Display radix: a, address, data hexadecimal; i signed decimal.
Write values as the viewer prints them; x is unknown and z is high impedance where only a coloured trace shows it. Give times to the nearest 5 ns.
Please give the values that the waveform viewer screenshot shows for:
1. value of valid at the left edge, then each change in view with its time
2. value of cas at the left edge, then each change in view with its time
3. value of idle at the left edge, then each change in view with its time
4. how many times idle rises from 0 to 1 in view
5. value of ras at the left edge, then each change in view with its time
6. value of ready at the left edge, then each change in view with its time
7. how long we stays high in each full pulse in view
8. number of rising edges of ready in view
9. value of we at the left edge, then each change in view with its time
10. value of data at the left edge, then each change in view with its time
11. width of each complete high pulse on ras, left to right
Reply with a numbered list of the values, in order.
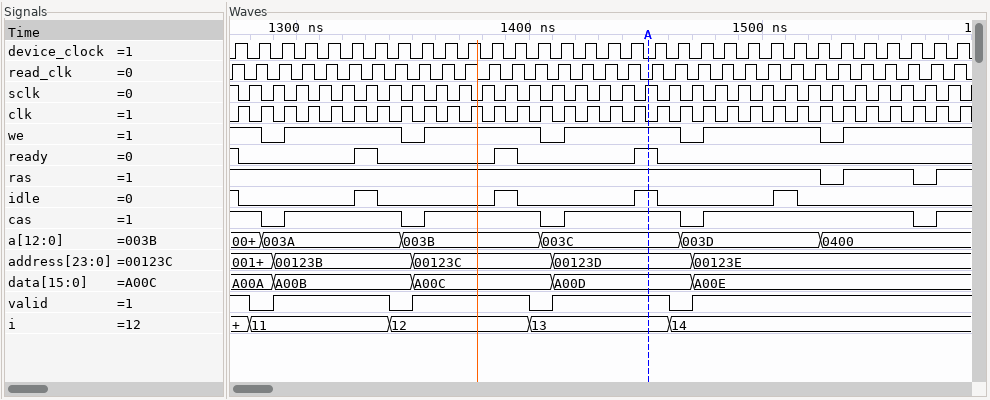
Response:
1. 1, 0 at 1280 ns, 1 at 1290 ns, 0 at 1340 ns, 1 at 1350 ns, 0 at 1400 ns, 1 at 1410 ns, 0 at 1460 ns, 1 at 1470 ns
2. 1, 0 at 1285 ns, 1 at 1295 ns, 0 at 1345 ns, 1 at 1355 ns, 0 at 1405 ns, 1 at 1415 ns, 0 at 1465 ns, 1 at 1475 ns, 0 at 1565 ns, 1 at 1575 ns
3. 1, 0 at 1275 ns, 1 at 1325 ns, 0 at 1335 ns, 1 at 1385 ns, 0 at 1395 ns, 1 at 1445 ns, 0 at 1455 ns, 1 at 1505 ns, 0 at 1515 ns
4. 4
5. 1, 0 at 1525 ns, 1 at 1535 ns, 0 at 1565 ns, 1 at 1575 ns
6. 1, 0 at 1275 ns, 1 at 1325 ns, 0 at 1335 ns, 1 at 1385 ns, 0 at 1395 ns, 1 at 1445 ns, 0 at 1455 ns
7. 50 ns, 50 ns, 50 ns, 50 ns
8. 3
9. 1, 0 at 1285 ns, 1 at 1295 ns, 0 at 1345 ns, 1 at 1355 ns, 0 at 1405 ns, 1 at 1415 ns, 0 at 1465 ns, 1 at 1475 ns, 0 at 1525 ns, 1 at 1535 ns
10. A00A, A00B at 1290 ns, A00C at 1350 ns, A00D at 1410 ns, A00E at 1470 ns
11. 30 ns
